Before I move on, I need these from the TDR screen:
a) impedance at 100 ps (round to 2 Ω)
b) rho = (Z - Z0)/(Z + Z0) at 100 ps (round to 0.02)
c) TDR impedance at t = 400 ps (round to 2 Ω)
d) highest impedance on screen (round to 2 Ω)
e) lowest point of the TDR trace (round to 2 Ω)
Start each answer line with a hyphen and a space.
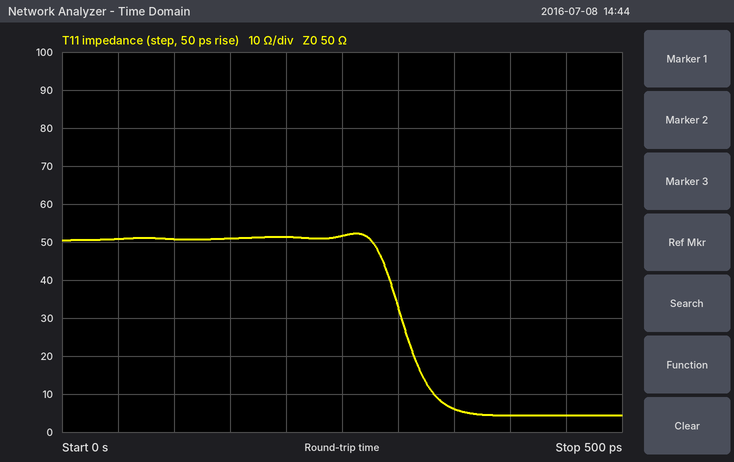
- 50 Ω
- 0.00
- 4 Ω
- 52 Ω
- 4 Ω
